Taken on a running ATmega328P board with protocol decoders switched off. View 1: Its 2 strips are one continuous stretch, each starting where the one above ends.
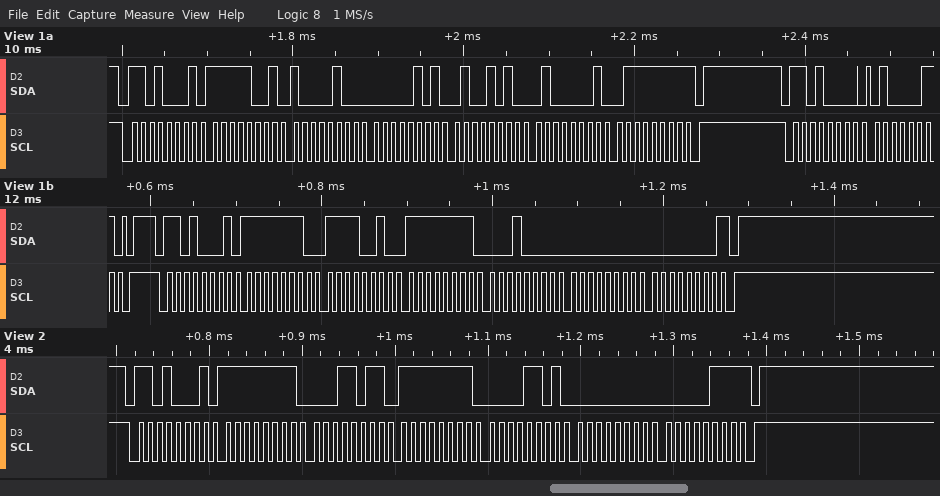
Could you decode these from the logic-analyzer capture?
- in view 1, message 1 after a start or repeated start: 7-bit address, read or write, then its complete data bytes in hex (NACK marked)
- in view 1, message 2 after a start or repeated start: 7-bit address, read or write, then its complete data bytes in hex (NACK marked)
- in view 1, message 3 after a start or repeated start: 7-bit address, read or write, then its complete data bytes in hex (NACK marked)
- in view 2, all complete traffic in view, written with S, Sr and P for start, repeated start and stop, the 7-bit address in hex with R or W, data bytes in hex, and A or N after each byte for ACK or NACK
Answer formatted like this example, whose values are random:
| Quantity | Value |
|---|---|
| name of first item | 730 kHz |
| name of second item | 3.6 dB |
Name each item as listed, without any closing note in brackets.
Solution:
| Quantity | Value |
|---|---|
| in view 1, message 1 after a start or repeated start: 7-bit address, read or write, then its complete data bytes in hex | 0x68 read: F9 84 05 4A 41 7F NACK |
| in view 1, message 2 after a start or repeated start: 7-bit address, read or write, then its complete data bytes in hex | 0x68 write: 43 |
| in view 1, message 3 after a start or repeated start: 7-bit address, read or write, then its complete data bytes in hex | 0x68 read: FE F2 FF 10 00 00 NACK |
| in view 2, all complete traffic in view, written with S, Sr and P for start, repeated start and stop, the 7-bit address in hex with R or W, data bytes in hex, and A or N after each byte for ACK or NACK | S 68R A FF A 1B A FF A 0D A 00 A 07 N P |
